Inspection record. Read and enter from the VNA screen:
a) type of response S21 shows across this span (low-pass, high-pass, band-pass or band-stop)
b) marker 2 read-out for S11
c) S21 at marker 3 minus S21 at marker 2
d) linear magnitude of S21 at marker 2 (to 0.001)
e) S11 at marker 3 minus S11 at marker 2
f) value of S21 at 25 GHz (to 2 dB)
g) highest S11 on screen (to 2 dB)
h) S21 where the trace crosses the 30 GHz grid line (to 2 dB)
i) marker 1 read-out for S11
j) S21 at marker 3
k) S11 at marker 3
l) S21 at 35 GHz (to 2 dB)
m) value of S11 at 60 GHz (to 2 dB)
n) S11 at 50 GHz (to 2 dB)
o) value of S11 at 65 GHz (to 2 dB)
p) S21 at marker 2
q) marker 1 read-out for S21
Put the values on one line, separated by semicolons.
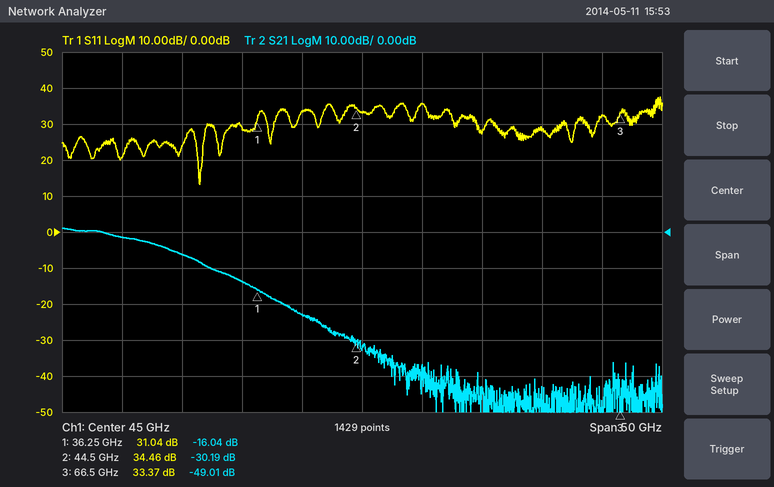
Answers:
low-pass; 34.46 dB; -18.82 dB; 0.031; -1.09 dB; -2 dB; 38 dB; -6 dB; 31.04 dB; -49.01 dB; 33.37 dB; -14 dB; 28 dB; 36 dB; 32 dB; -30.19 dB; -16.04 dB
